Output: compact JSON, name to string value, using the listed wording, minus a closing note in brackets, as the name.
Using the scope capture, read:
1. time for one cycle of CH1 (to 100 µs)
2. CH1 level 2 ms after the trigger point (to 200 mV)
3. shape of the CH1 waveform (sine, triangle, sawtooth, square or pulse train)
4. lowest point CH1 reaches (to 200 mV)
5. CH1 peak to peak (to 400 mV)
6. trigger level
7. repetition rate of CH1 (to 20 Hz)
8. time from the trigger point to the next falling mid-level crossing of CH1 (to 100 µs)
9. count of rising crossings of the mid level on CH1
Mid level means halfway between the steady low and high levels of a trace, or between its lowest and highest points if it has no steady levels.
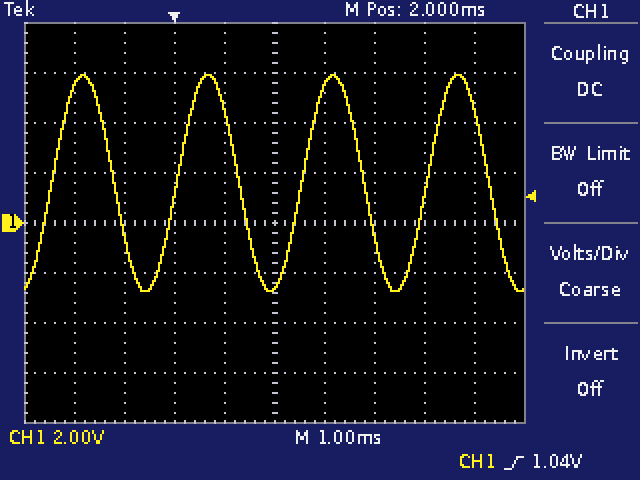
{"time for one cycle of CH1": "2.5 ms", "CH1 level 2 ms after the trigger point": "-2.6 V", "shape of the CH1 waveform": "sine", "lowest point CH1 reaches": "-2.8 V", "CH1 peak to peak": "8.8 V", "trigger level": "1.04 V", "repetition rate of CH1": "400 Hz", "time from the trigger point to the next falling mid-level crossing of CH1": "1.3 ms", "count of rising crossings of the mid level on CH1": "4"}
